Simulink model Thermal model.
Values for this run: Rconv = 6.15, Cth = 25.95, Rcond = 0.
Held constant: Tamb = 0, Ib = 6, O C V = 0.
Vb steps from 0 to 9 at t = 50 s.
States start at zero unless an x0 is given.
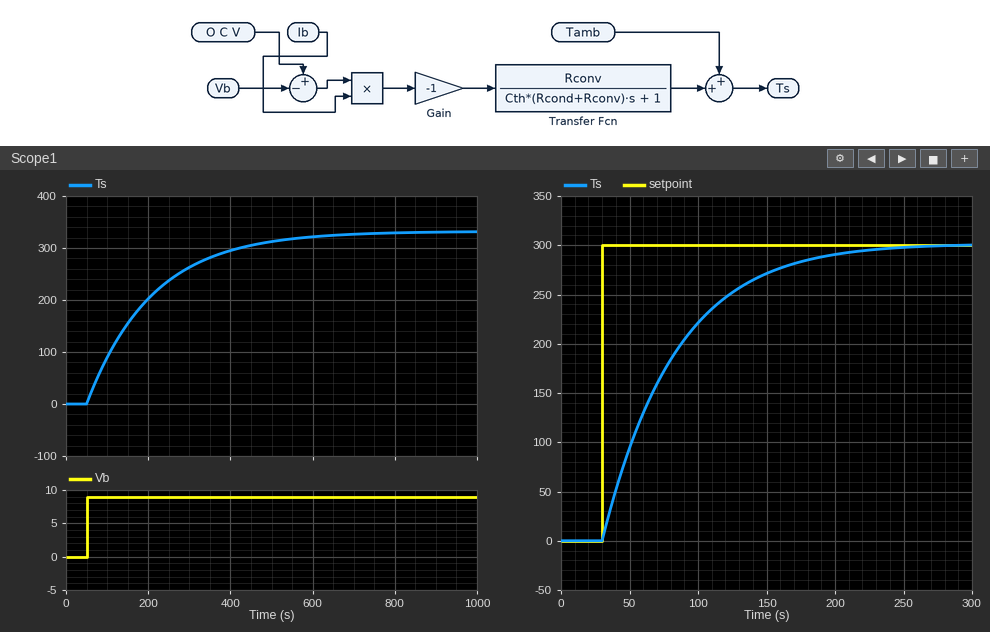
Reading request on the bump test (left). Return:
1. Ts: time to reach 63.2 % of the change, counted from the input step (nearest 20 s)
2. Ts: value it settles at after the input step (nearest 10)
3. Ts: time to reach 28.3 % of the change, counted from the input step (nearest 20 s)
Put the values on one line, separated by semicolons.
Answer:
160 s; 330; 60 s
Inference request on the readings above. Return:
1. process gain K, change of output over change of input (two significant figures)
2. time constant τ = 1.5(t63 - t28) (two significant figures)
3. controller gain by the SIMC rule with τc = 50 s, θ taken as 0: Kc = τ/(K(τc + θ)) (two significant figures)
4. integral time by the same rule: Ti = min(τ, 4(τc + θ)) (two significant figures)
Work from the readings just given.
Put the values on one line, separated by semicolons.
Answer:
37; 150 s; 0.081; 150 s
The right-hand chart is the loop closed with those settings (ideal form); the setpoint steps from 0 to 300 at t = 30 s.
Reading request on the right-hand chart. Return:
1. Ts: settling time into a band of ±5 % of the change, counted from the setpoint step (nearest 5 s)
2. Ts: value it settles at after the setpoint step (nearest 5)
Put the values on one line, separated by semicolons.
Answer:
150 s; 300
